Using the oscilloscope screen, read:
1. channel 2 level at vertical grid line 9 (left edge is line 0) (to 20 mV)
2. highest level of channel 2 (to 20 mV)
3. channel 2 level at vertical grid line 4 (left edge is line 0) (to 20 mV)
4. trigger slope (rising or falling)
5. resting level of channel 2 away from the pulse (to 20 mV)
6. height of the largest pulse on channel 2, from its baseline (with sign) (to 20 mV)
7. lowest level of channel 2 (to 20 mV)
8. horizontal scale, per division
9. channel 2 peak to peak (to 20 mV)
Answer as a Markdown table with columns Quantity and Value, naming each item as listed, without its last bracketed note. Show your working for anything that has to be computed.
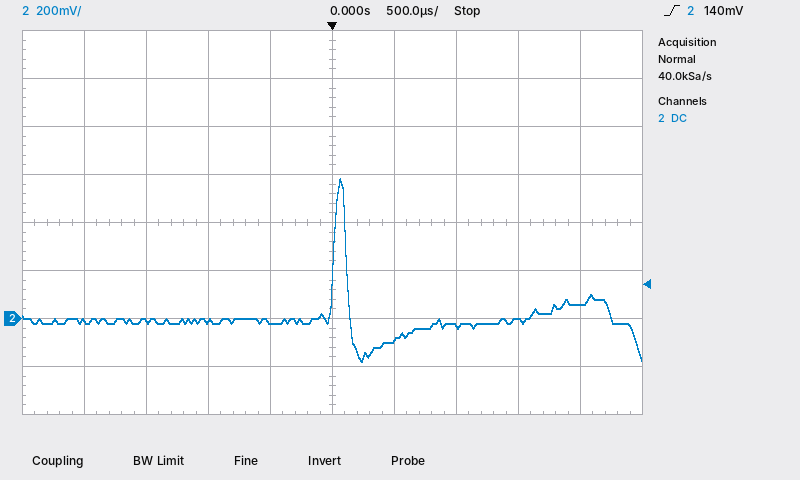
| Quantity | Value |
|---|---|
| channel 2 level at vertical grid line 9 (left edge is line 0) | 60 mV |
| highest level of channel 2 | 580 mV |
| channel 2 level at vertical grid line 4 (left edge is line 0) | -20 mV |
| trigger slope | rising |
| resting level of channel 2 away from the pulse | -20 mV |
| height of the largest pulse on channel 2, from its baseline (with sign) | 580 mV − (-20 mV) = +600 mV |
| lowest level of channel 2 | -180 mV |
| horizontal scale, per division | 500 µs |
| channel 2 peak to peak | 580 mV − (-180 mV) = 760 mV |
